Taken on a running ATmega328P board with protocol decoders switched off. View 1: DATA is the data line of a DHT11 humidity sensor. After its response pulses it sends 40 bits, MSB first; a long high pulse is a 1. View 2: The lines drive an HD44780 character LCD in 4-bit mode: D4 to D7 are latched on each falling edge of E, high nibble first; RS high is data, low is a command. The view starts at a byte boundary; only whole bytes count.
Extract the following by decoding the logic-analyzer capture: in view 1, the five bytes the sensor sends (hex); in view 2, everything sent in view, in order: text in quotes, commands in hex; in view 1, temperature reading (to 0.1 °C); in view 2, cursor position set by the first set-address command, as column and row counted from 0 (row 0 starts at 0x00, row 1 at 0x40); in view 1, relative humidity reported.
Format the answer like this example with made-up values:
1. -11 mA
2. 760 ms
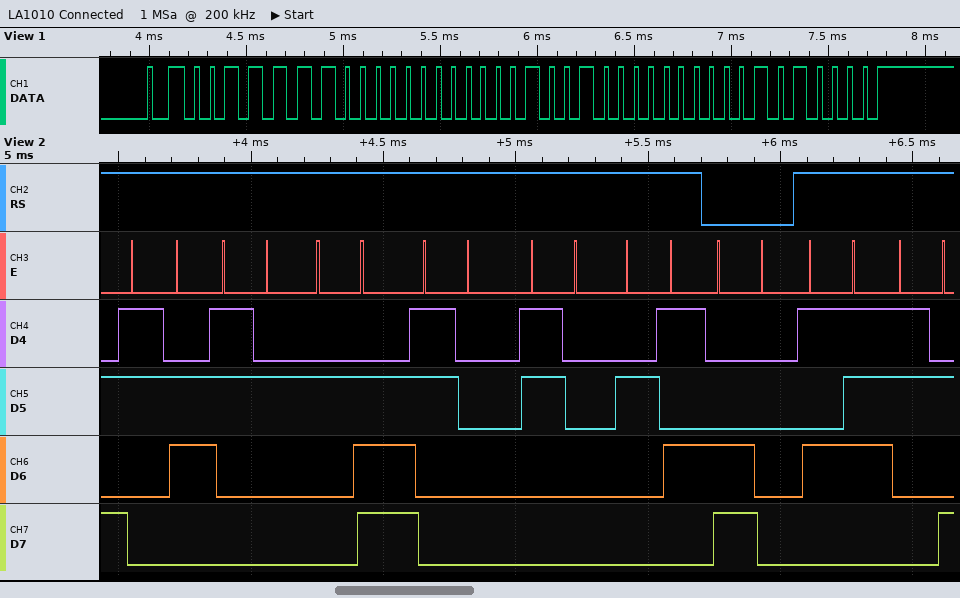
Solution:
1. 3E 00 12 00 50
2. "62.00%" 0xC0 "W:"
3. 18.0 °C
4. column 0, row 1
5. 62 %
